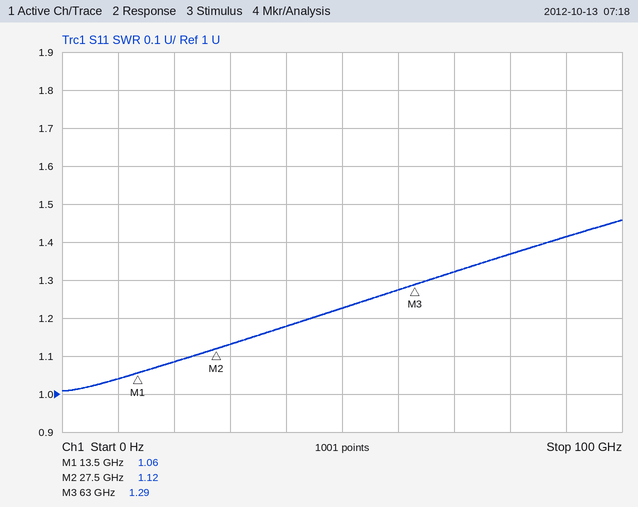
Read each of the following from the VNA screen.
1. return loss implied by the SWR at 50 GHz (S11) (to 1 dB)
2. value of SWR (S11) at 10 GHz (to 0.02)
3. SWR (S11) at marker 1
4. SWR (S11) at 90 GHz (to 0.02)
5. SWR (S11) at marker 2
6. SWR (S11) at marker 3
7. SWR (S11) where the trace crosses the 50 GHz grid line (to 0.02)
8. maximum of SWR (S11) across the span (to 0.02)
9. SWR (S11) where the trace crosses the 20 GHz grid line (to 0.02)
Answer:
20 dB
1.04
1.06
1.42
1.12
1.29
1.22
1.46
1.08
